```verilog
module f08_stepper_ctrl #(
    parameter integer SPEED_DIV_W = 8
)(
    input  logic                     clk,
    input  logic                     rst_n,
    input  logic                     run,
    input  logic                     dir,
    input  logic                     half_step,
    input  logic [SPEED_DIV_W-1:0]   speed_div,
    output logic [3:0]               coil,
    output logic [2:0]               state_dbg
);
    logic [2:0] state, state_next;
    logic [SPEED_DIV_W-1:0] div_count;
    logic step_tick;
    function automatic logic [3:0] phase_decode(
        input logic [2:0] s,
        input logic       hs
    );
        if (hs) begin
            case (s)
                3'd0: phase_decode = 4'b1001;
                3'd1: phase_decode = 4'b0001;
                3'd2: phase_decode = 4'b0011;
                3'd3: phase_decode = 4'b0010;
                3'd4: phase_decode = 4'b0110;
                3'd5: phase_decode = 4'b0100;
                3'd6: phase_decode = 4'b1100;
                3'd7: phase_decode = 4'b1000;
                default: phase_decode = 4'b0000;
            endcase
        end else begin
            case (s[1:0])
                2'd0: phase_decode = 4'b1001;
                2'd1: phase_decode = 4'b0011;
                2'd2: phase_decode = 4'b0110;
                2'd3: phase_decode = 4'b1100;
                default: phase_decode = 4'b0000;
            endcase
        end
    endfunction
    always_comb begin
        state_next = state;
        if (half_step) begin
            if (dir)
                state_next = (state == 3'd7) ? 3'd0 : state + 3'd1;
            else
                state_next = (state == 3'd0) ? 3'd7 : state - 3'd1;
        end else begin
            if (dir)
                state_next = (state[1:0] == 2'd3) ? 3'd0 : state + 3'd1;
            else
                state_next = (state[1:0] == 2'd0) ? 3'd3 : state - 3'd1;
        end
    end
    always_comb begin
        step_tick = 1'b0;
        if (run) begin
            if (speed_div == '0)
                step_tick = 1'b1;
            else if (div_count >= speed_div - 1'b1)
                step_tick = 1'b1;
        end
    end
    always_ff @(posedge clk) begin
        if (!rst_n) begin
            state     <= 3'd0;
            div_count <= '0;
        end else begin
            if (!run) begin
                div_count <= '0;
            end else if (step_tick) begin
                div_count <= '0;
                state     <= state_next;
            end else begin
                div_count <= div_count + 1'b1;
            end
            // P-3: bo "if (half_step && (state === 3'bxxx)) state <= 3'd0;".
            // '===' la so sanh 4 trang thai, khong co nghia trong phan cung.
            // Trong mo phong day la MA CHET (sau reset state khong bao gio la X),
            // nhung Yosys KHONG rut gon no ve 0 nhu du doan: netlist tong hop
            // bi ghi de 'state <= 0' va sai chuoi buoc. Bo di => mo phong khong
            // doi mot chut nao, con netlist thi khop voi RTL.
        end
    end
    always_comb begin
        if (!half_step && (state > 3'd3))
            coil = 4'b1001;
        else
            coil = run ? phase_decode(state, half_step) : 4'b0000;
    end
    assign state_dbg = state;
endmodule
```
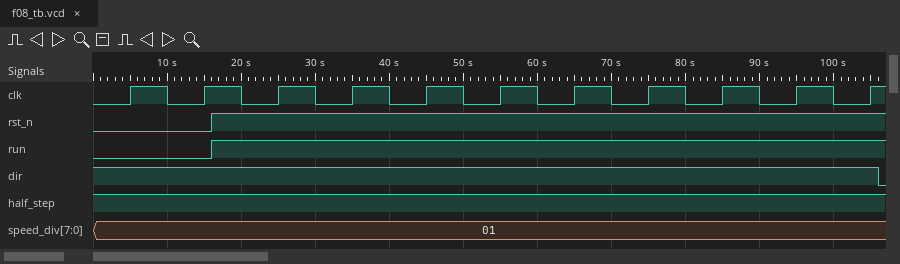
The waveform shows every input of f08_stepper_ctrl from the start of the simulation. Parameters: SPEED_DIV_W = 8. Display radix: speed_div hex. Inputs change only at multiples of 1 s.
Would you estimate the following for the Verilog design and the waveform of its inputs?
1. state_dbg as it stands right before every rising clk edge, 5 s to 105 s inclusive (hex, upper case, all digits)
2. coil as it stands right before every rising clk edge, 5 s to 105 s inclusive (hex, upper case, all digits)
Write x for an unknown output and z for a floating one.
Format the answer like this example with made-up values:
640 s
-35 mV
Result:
x, 0, 0, 1, 2, 3, 4, 5, 6, 7, 0
0, 0, 9, 1, 3, 2, 6, 4, C, 8, 9
